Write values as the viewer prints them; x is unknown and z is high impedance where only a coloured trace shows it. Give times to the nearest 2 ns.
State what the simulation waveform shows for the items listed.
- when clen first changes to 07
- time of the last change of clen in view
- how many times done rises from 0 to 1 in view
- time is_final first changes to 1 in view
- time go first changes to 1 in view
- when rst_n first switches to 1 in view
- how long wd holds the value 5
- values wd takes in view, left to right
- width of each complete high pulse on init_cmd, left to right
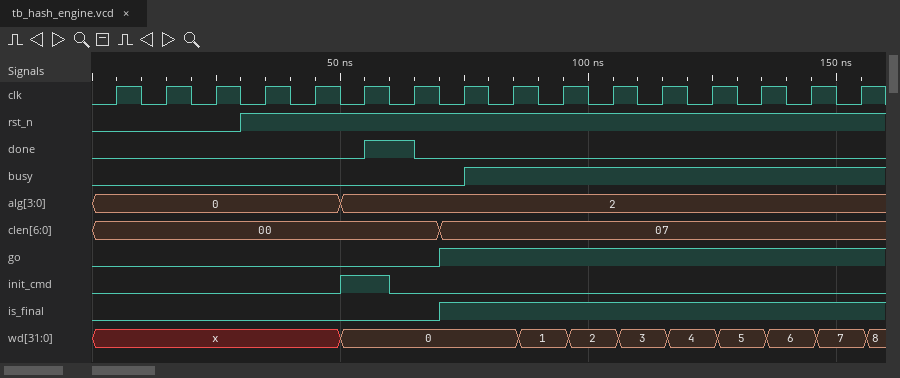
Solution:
70 ns
70 ns
1
70 ns
70 ns
30 ns
10 ns
x, 0, 1, 2, 3, 4, 5, 6, 7, 8
10 ns
